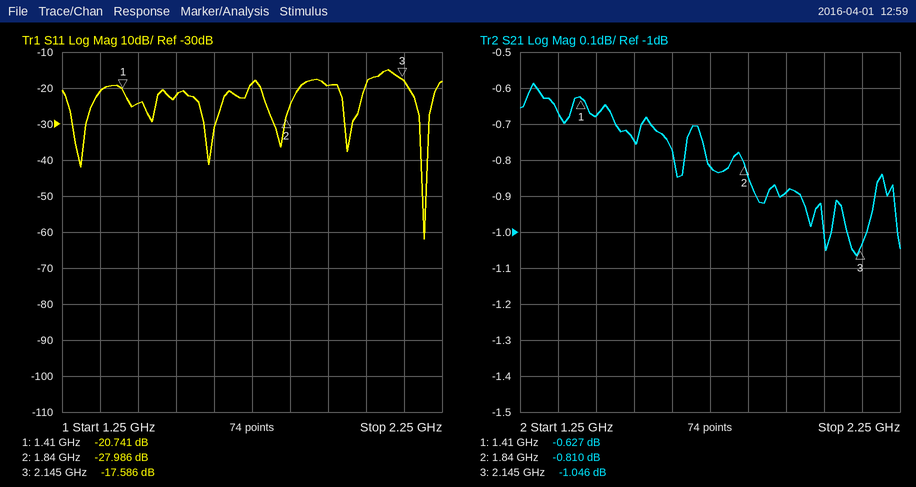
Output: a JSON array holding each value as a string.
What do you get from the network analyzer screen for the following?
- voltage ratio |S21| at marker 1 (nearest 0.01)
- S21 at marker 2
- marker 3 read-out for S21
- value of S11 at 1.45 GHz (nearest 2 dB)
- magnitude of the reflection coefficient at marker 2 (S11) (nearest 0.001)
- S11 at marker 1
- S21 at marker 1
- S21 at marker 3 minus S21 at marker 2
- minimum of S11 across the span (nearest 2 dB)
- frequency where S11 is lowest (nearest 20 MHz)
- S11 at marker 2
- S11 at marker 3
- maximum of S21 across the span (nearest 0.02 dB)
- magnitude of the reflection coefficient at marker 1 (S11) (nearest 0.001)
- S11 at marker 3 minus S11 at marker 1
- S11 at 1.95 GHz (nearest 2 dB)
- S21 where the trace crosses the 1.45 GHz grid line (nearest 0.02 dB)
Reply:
["0.93", "-0.810 dB", "-1.046 dB", "-24 dB", "0.040", "-20.741 dB", "-0.627 dB", "-0.236 dB", "-62 dB", "2.20 GHz", "-27.986 dB", "-17.586 dB", "-0.58 dB", "0.092", "3.155 dB", "-20 dB", "-0.68 dB"]
